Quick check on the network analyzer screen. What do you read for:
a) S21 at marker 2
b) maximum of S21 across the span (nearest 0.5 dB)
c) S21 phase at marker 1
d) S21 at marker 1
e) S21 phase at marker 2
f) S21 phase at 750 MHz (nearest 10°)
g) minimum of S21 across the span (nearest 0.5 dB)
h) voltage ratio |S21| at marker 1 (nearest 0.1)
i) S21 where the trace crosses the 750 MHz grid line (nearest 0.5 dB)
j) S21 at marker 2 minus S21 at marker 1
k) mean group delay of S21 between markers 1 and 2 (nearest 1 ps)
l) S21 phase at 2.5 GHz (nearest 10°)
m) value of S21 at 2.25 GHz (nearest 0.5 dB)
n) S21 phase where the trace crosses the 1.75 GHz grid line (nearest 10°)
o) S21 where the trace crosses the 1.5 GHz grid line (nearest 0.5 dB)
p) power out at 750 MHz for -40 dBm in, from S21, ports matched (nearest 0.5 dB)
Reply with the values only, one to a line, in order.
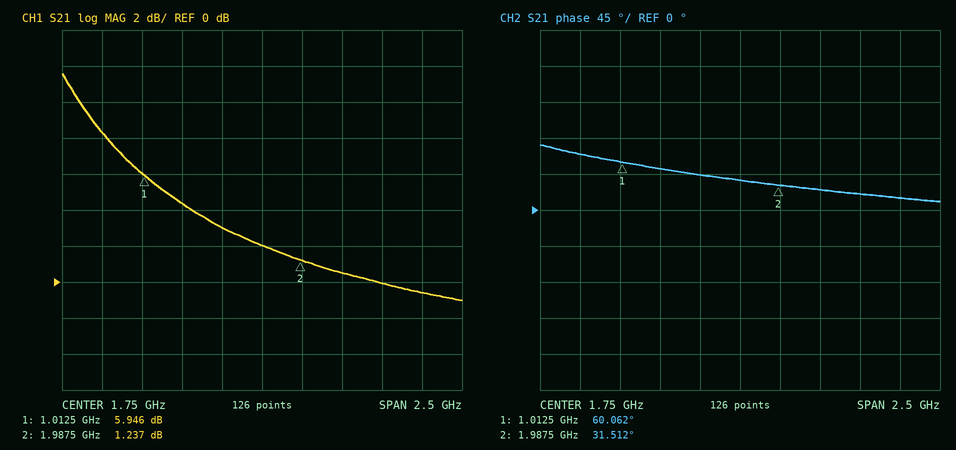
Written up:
1.237 dB
11.5 dB
60.062°
5.946 dB
31.512°
70°
-1.0 dB
2.0
8.5 dB
-4.709 dB
81 ps
20°
0.5 dB
40°
3.0 dB
-31.5 dBm
